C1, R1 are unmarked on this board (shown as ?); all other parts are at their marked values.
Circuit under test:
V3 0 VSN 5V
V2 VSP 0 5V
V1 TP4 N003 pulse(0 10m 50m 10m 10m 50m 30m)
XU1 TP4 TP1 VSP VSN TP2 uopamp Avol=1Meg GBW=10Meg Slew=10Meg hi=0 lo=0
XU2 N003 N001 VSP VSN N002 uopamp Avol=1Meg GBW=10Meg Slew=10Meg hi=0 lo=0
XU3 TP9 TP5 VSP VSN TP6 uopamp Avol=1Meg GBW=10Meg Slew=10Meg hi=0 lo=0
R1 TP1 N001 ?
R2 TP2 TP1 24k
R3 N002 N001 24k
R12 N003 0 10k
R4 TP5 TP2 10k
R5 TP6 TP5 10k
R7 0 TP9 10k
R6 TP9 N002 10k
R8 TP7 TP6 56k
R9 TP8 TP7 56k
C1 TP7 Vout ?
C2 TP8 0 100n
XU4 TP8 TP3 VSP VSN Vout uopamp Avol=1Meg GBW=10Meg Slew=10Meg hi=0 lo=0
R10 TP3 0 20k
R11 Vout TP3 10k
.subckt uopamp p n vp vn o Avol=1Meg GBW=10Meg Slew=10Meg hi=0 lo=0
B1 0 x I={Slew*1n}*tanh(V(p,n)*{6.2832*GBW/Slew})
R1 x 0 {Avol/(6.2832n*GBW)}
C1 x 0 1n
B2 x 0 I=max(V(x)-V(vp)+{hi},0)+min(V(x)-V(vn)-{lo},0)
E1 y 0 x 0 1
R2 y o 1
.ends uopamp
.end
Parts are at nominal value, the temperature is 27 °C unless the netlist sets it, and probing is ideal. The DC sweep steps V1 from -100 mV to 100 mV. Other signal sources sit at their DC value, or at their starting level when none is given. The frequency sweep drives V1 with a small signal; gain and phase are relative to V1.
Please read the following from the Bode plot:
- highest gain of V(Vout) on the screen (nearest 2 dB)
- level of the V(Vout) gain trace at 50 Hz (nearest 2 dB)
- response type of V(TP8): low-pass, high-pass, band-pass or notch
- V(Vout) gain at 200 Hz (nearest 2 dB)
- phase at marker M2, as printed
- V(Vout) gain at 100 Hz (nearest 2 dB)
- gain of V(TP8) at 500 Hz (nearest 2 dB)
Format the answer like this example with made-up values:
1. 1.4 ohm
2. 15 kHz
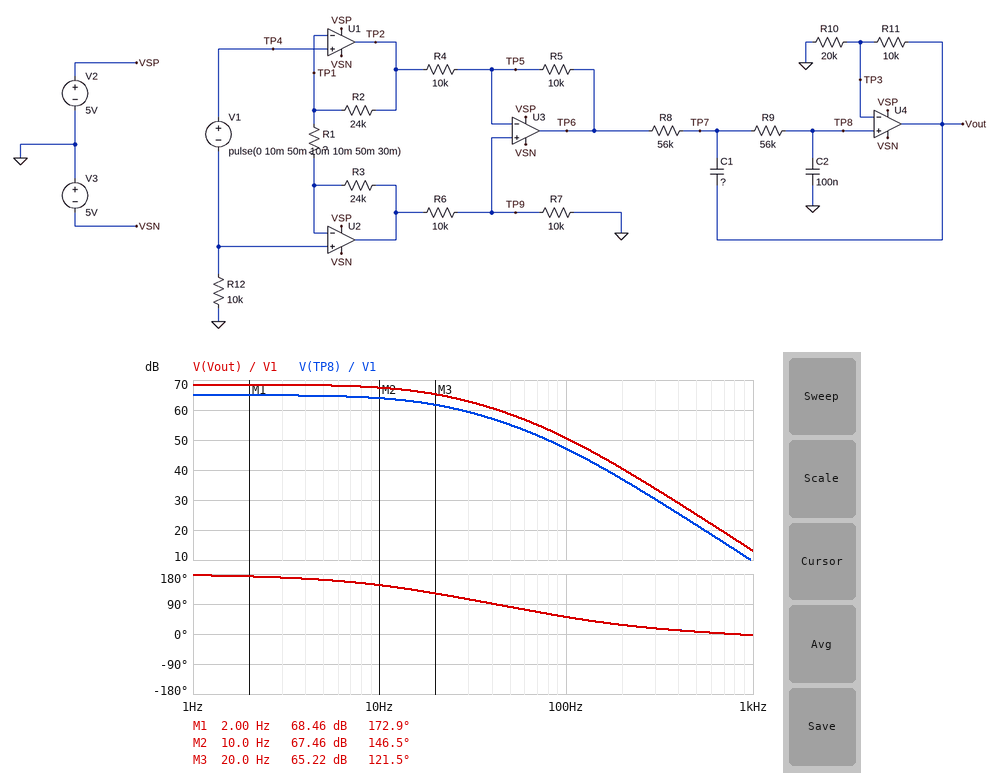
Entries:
1. 68 dB
2. 58 dB
3. low-pass
4. 40 dB
5. 146.5 deg
6. 50 dB
7. 22 dB
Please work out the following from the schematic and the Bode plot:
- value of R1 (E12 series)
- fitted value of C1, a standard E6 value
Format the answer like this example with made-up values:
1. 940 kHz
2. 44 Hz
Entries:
1. 27 Ω
2. 47 nF
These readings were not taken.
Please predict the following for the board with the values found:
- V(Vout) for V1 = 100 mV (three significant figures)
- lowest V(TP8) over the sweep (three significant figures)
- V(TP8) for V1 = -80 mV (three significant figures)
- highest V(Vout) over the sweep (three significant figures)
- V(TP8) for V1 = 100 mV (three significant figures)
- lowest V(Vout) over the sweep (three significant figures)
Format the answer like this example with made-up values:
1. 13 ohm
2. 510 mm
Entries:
1. -5.01 V
2. -5.01 V
3. 5.01 V
4. 5.01 V
5. -5.01 V
6. -5.01 V
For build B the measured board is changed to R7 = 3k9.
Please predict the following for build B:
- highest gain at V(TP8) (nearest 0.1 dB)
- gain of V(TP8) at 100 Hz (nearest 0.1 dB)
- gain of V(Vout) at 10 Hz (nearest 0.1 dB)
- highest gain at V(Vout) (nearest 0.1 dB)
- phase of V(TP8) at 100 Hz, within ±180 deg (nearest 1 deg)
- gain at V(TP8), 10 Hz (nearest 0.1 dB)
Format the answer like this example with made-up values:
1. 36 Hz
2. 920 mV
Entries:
1. 62.8 dB
2. 44.9 dB
3. 65.3 dB
4. 66.4 dB
5. 51 deg
6. 61.8 dB
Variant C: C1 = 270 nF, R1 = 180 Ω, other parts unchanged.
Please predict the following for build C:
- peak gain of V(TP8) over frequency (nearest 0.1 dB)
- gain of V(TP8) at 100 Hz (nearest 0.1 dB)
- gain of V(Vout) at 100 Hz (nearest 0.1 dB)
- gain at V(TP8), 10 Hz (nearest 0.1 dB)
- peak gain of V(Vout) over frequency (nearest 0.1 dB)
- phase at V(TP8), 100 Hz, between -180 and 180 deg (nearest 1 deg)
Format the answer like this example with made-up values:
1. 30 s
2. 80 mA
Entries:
1. 56.8 dB
2. 18.3 dB
3. 21.8 dB
4. 51.6 dB
5. 60.3 dB
6. 4 deg
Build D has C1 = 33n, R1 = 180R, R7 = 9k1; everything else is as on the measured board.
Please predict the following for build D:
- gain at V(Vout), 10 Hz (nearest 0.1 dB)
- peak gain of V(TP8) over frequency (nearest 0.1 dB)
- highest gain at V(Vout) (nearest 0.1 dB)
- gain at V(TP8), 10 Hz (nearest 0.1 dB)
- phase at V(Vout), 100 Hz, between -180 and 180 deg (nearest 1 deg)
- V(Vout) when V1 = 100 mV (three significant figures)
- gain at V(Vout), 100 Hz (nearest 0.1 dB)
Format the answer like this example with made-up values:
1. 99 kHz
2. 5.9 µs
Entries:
1. 50.6 dB
2. 48.3 dB
3. 51.9 dB
4. 47.1 dB
5. 64 deg
6. -5.01 V
7. 34.8 dB
